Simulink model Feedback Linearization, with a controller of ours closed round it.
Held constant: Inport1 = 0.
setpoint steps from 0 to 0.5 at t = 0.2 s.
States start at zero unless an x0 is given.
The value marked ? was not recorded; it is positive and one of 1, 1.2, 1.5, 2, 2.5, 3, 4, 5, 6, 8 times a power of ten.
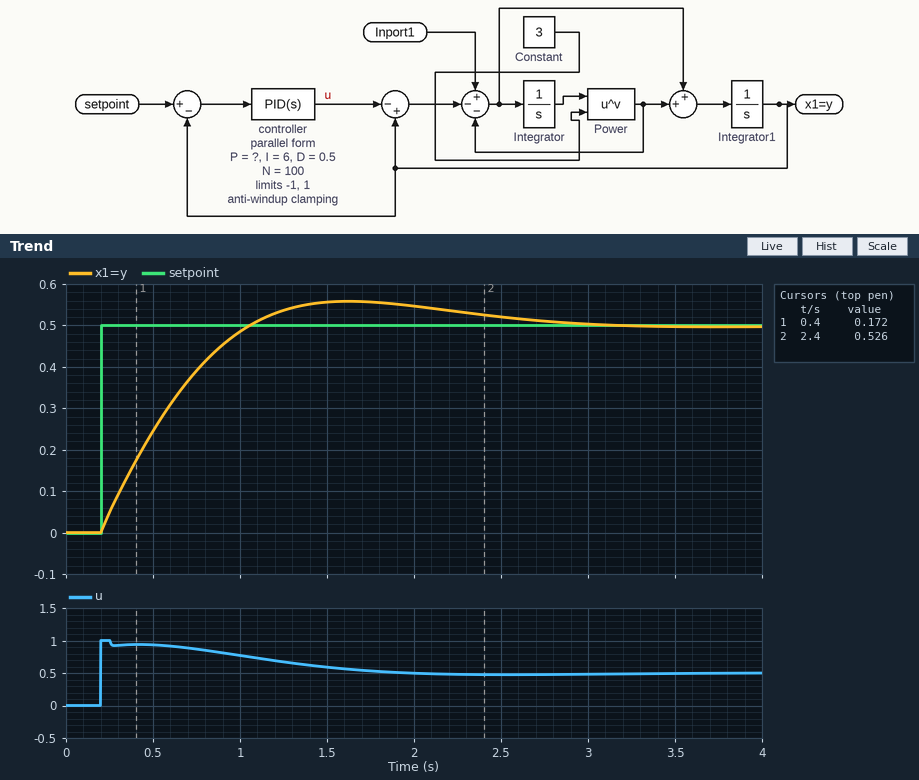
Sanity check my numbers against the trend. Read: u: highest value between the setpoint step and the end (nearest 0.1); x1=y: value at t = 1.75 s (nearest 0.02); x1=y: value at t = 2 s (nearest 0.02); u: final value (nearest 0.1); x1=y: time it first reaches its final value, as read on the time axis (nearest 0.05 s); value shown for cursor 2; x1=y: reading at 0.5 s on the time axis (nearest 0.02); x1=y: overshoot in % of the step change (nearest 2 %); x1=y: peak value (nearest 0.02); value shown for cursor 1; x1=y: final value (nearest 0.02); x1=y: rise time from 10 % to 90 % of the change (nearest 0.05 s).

1.0
0.56
0.54
0.5
1.05 s
0.526
0.24
12 %
0.56
0.172
0.50
0.65 s
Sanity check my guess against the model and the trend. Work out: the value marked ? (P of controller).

3
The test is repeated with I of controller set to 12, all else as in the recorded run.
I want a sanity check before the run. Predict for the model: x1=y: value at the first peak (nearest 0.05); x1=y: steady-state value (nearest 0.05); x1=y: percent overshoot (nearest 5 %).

0.60
0.50
15 %
